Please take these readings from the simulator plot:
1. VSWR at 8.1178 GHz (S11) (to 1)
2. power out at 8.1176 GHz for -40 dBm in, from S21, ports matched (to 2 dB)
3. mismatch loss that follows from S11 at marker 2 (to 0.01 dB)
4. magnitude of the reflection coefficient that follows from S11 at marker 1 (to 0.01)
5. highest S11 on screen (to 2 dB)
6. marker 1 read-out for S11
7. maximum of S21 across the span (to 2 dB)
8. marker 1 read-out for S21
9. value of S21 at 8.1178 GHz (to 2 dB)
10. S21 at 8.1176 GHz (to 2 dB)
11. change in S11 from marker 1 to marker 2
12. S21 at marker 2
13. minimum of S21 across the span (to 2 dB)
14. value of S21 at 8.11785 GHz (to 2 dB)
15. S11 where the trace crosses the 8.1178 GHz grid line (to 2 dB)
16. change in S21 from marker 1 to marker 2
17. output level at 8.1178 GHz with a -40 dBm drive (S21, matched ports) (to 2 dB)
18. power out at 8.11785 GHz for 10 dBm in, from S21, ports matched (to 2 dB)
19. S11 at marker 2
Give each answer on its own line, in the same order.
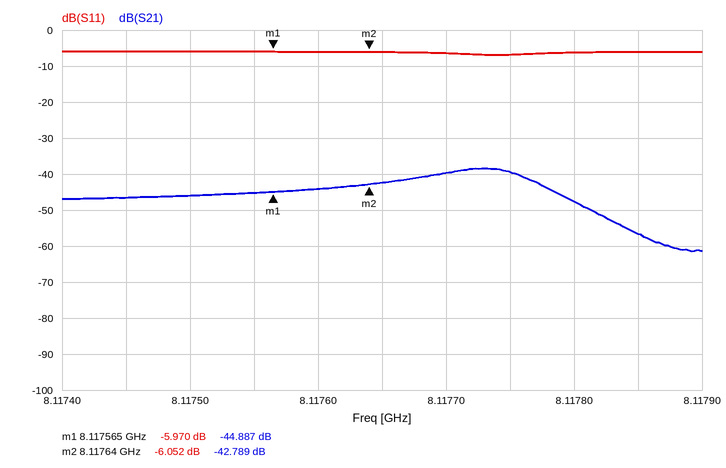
3
-84 dBm
1.24 dB
0.50
-6 dB
-5.970 dB
-38 dB
-44.887 dB
-48 dB
-44 dB
-0.082 dB
-42.789 dB
-62 dB
-56 dB
-6 dB
2.098 dB
-88 dBm
-46 dBm
-6.052 dB
